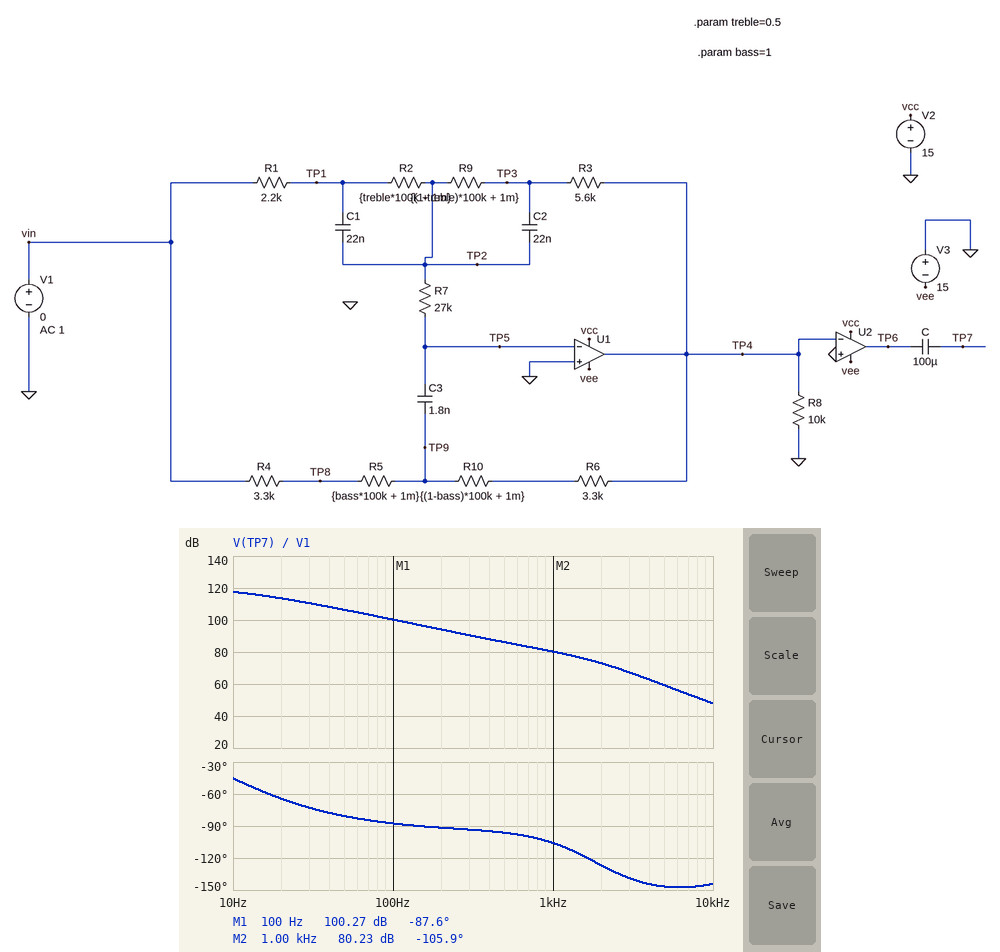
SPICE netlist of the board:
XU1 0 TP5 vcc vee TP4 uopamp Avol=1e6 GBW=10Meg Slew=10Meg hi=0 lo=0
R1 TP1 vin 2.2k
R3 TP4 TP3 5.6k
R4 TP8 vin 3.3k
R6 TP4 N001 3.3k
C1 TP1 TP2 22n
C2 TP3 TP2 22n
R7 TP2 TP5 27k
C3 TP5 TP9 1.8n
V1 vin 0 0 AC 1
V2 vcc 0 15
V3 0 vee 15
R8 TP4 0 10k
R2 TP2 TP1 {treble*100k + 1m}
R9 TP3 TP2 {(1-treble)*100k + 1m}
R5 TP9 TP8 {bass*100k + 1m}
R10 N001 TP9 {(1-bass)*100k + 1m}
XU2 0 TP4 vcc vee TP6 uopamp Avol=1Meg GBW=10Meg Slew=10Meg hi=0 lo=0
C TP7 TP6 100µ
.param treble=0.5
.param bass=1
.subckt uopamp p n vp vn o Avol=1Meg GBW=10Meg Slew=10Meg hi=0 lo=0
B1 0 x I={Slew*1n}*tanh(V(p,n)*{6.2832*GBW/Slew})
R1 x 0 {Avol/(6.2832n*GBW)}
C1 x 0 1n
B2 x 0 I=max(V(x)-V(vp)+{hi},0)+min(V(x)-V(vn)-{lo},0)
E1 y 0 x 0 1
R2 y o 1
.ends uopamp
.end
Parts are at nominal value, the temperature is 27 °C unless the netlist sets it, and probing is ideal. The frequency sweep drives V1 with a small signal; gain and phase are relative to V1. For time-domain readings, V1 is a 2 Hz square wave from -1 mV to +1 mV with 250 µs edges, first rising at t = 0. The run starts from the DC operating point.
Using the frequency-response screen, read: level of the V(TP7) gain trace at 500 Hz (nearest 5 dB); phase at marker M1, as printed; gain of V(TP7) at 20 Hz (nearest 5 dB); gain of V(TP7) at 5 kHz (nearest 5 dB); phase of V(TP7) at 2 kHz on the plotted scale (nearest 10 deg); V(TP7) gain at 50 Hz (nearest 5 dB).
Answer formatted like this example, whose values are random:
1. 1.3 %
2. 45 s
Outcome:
1. 85 dB
2. -87.6 deg
3. 115 dB
4. 60 dB
5. -130 deg
6. 105 dB
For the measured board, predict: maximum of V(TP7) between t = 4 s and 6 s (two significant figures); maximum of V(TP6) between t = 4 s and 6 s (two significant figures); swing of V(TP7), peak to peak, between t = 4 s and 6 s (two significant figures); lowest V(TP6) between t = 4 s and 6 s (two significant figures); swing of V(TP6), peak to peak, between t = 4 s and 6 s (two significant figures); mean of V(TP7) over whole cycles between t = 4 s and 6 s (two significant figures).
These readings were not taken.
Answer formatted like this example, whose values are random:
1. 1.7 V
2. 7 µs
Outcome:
1. 30 V
2. 15 V
3. 30 V
4. -15 V
5. 30 V
6. 15 V
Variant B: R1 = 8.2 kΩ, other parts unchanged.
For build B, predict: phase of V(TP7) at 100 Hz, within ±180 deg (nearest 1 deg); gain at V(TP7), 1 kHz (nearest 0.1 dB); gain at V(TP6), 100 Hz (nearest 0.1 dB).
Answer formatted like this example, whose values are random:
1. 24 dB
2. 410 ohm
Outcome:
1. -91 deg
2. 76.2 dB
3. 99.3 dB
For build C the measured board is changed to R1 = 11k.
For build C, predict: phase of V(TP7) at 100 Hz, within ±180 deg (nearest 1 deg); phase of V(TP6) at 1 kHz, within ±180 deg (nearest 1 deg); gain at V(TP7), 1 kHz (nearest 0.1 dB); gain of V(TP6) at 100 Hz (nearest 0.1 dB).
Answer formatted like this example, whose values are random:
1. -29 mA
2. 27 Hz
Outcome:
1. -93 deg
2. -130 deg
3. 74.7 dB
4. 98.8 dB
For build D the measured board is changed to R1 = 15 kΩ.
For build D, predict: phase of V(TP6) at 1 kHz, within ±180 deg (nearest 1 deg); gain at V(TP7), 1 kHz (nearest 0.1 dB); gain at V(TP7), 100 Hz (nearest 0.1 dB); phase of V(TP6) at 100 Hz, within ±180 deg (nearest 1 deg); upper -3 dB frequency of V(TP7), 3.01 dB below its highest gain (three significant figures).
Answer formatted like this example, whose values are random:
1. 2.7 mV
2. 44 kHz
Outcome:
1. -135 deg
2. 72.8 dB
3. 98.2 dB
4. -95 deg
5. 9.99 Hz
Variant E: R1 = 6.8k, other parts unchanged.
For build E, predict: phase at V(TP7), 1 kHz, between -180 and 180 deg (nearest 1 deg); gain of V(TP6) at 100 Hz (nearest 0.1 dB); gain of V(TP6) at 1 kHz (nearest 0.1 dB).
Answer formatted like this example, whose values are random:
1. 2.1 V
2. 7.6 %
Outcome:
1. -122 deg
2. 99.5 dB
3. 77.1 dB
